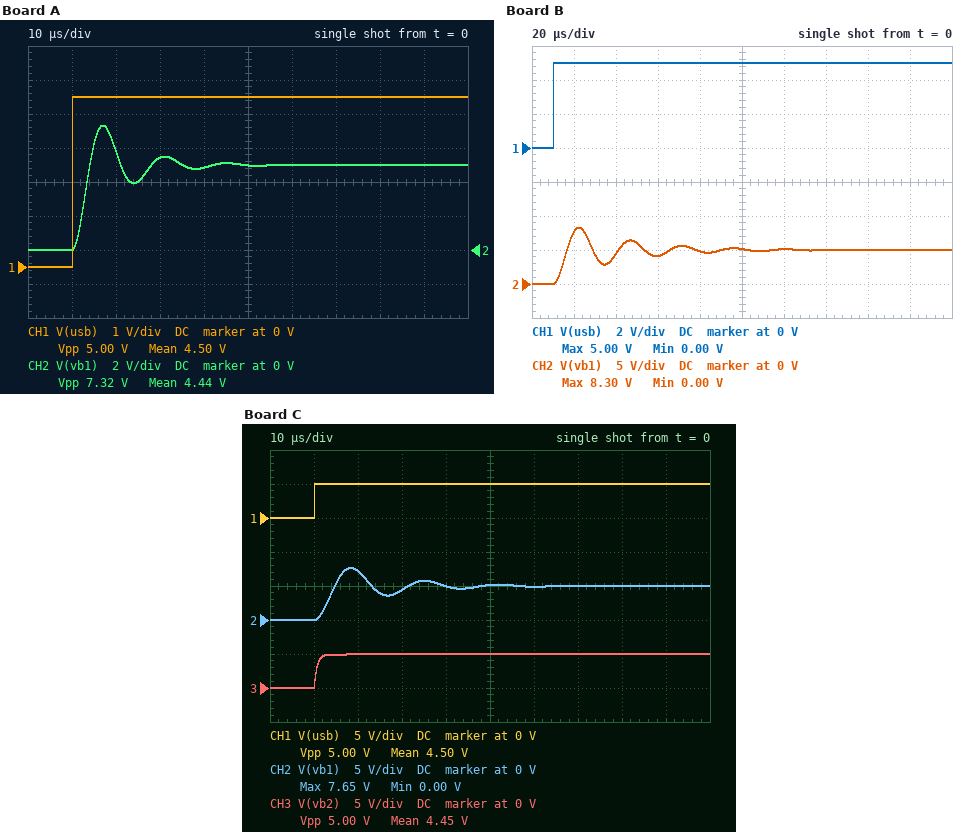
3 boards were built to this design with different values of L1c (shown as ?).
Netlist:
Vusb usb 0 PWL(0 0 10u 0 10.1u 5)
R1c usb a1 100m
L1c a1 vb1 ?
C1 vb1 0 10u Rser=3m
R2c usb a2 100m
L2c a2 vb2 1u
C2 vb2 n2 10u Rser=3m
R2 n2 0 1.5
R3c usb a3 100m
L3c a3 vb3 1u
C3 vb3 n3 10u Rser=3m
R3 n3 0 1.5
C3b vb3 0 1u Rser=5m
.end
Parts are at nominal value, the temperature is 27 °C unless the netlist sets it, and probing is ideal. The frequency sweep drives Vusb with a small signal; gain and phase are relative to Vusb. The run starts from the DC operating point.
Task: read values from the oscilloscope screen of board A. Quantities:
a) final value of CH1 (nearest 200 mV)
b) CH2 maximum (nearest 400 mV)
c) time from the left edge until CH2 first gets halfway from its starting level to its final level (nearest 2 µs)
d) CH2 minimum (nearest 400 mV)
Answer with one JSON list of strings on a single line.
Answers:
["5.0 V", "7.2 V", "12 µs", "0 V"]
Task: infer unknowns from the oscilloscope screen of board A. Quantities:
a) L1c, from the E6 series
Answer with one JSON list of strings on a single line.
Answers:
["470 nH"]
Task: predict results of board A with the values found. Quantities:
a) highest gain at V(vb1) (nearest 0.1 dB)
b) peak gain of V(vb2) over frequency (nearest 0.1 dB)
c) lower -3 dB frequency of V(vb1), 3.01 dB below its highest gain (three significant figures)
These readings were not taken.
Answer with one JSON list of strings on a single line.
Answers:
["6.7 dB", "0 dB", "47.9 kHz"]
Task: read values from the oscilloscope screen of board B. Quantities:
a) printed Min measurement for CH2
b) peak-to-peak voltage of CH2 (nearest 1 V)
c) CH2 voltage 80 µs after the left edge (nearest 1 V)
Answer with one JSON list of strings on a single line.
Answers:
["0.00 V", "8 V", "5 V"]
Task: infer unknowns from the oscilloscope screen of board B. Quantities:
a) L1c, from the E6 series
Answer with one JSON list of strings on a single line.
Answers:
["1.5 µH"]
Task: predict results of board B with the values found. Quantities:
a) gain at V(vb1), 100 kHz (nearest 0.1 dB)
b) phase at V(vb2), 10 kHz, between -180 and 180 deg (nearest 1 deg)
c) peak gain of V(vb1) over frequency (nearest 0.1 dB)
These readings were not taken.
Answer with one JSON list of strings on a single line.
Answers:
["-13.9 dB", "-3 deg", "11.6 dB"]
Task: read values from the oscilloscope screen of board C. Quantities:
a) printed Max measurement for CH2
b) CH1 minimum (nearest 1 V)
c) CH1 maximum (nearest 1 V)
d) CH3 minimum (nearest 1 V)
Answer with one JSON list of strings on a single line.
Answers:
["7.65 V", "0 V", "5 V", "0 V"]
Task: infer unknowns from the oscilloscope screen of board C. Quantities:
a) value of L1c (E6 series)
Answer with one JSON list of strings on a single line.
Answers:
["680 nH"]
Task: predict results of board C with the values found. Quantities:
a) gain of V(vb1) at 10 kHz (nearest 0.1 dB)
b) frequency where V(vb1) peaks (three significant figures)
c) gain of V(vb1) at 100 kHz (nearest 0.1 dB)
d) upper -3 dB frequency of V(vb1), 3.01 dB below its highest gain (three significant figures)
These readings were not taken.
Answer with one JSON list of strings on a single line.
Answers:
["0.2 dB", "58.6 kHz", "-5.1 dB", "69.8 kHz"]
